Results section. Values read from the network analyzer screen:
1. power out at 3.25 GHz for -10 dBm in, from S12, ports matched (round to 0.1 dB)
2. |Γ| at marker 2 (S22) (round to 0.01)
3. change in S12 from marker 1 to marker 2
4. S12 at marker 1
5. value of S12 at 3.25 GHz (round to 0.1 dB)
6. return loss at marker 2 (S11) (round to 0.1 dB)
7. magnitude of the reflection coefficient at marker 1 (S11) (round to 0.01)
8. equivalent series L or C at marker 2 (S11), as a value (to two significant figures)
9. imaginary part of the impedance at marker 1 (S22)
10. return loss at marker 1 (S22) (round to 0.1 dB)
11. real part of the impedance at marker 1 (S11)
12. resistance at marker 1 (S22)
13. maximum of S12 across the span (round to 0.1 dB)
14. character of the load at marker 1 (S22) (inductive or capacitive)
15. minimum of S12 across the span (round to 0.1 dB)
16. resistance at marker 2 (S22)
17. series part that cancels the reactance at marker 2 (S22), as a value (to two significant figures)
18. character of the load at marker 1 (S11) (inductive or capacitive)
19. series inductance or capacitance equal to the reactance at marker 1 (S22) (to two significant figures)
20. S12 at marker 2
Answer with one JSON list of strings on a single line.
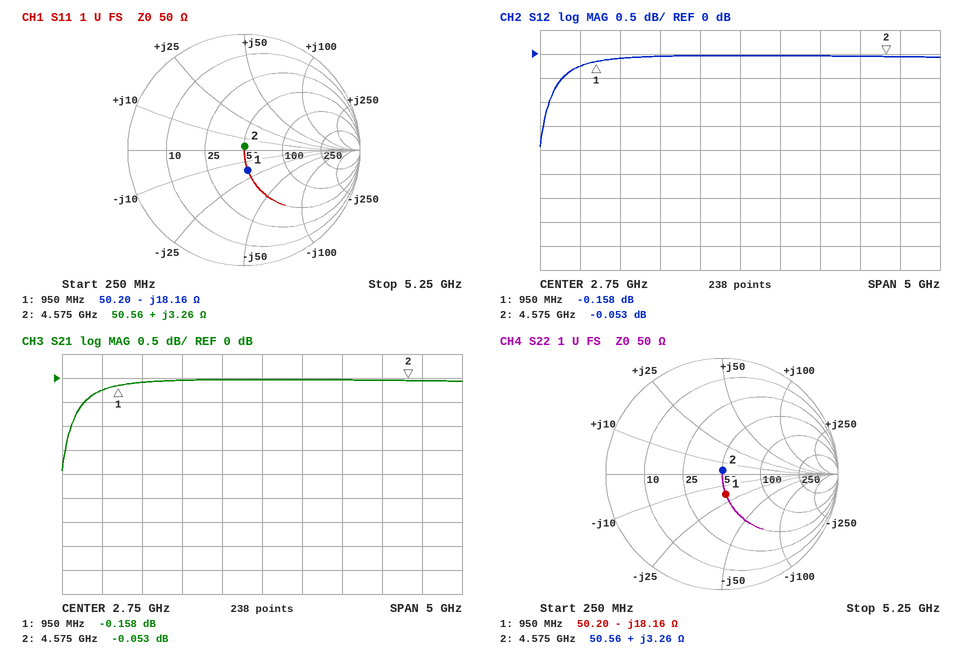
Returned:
["-10.0 dBm", "0.03", "0.105 dB", "-0.158 dB", "0.0 dB", "29.7 dB", "0.18", "110 pH", "-18.16 Ω", "15.0 dB", "50.20 Ω", "50.20 Ω", "0.0 dB", "capacitive", "-1.9 dB", "50.56 Ω", "11 pF", "capacitive", "9.2 pF", "-0.053 dB"]
